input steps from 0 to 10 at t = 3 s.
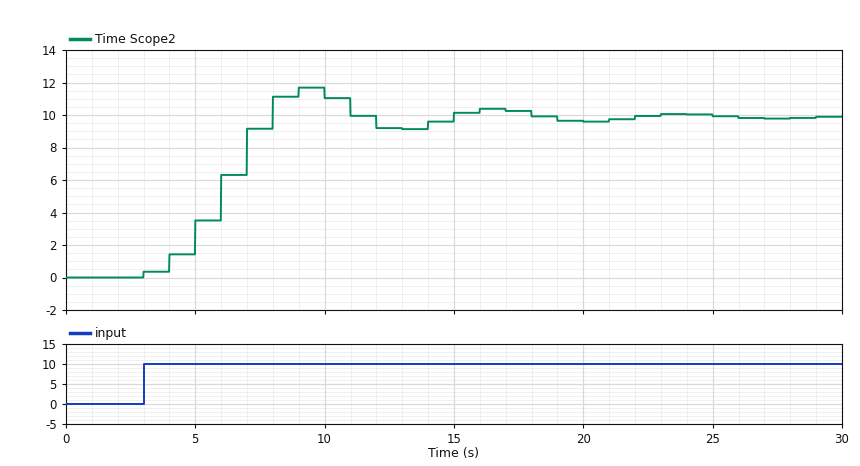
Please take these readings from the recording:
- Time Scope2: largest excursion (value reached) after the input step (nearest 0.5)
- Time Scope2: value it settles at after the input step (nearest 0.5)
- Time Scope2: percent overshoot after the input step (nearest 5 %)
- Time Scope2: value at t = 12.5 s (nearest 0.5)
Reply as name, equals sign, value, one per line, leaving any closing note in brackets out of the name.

Time Scope2: largest excursion (value reached) after the input step = 11.5
Time Scope2: value it settles at after the input step = 10.0
Time Scope2: percent overshoot after the input step = 20 %
Time Scope2: value at t = 12.5 s = 9.0
